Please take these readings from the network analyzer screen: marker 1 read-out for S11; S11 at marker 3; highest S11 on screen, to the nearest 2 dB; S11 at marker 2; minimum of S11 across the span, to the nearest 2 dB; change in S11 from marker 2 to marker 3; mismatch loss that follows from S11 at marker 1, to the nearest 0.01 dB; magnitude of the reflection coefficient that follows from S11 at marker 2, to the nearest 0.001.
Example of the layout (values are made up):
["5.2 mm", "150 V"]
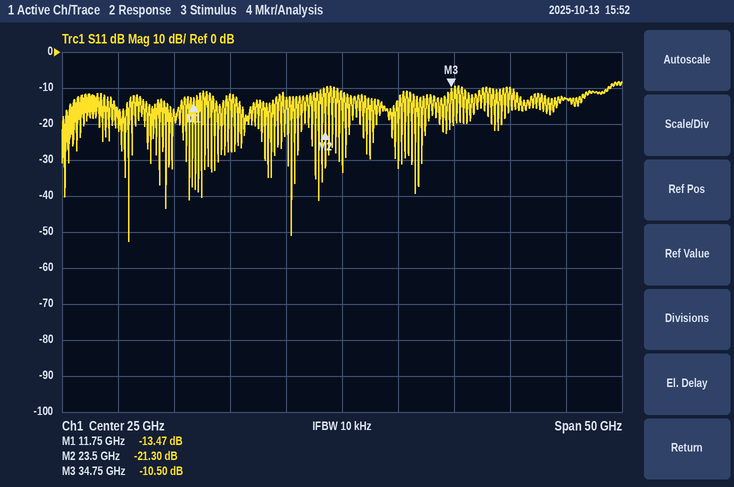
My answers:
["-13.47 dB", "-10.50 dB", "-8 dB", "-21.30 dB", "-52 dB", "10.80 dB", "0.20 dB", "0.086"]
